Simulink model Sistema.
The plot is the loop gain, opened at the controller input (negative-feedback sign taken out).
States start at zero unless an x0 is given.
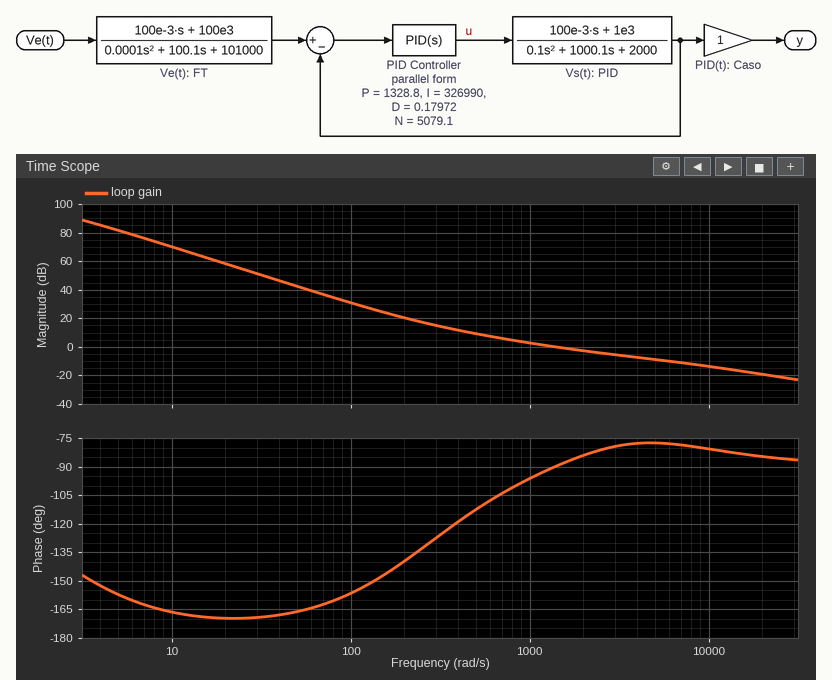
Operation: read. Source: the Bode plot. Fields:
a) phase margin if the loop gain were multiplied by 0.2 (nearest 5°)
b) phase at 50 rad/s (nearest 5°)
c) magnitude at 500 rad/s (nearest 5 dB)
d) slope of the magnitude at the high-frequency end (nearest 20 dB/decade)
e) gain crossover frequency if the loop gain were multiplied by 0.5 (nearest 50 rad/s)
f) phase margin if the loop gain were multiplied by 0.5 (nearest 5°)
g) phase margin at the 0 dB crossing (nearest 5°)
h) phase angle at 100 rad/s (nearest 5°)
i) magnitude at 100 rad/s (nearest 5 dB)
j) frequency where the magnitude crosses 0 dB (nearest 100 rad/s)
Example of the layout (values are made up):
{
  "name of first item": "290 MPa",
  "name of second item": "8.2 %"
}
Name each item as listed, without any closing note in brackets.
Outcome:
{
  "phase margin if the loop gain were multiplied by 0.2": "55°",
  "phase at 50 rad/s": "-165°",
  "magnitude at 500 rad/s": "10 dB",
  "slope of the magnitude at the high-frequency end": "-20 dB/decade",
  "gain crossover frequency if the loop gain were multiplied by 0.5": "700 rad/s",
  "phase margin if the loop gain were multiplied by 0.5": "75°",
  "phase margin at the 0 dB crossing": "90°",
  "phase angle at 100 rad/s": "-155°",
  "magnitude at 100 rad/s": "30 dB",
  "frequency where the magnitude crosses 0 dB": "1400 rad/s"
}
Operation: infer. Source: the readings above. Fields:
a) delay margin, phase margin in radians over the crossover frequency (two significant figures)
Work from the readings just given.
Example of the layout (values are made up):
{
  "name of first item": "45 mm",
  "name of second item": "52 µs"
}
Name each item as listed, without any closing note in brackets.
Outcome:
{
  "delay margin, phase margin in radians over the crossover frequency": "0.0011 s"
}
